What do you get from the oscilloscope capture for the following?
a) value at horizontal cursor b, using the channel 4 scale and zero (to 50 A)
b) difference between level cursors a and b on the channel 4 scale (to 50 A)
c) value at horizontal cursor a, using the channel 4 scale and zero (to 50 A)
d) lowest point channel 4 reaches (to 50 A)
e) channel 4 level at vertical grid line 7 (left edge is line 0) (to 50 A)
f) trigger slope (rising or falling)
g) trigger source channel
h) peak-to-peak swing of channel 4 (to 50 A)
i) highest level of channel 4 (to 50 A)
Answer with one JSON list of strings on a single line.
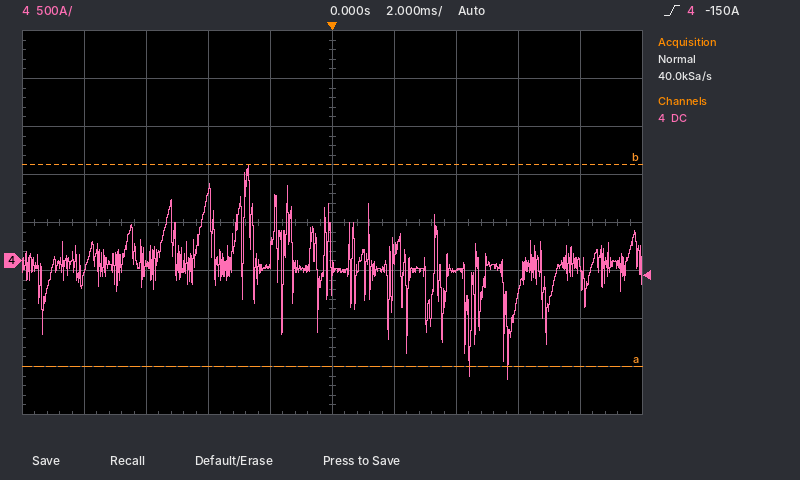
["1.00 kA", "2.10 kA", "-1.10 kA", "-1.25 kA", "-100 A", "rising", "channel 4", "2.25 kA", "1.00 kA"]
